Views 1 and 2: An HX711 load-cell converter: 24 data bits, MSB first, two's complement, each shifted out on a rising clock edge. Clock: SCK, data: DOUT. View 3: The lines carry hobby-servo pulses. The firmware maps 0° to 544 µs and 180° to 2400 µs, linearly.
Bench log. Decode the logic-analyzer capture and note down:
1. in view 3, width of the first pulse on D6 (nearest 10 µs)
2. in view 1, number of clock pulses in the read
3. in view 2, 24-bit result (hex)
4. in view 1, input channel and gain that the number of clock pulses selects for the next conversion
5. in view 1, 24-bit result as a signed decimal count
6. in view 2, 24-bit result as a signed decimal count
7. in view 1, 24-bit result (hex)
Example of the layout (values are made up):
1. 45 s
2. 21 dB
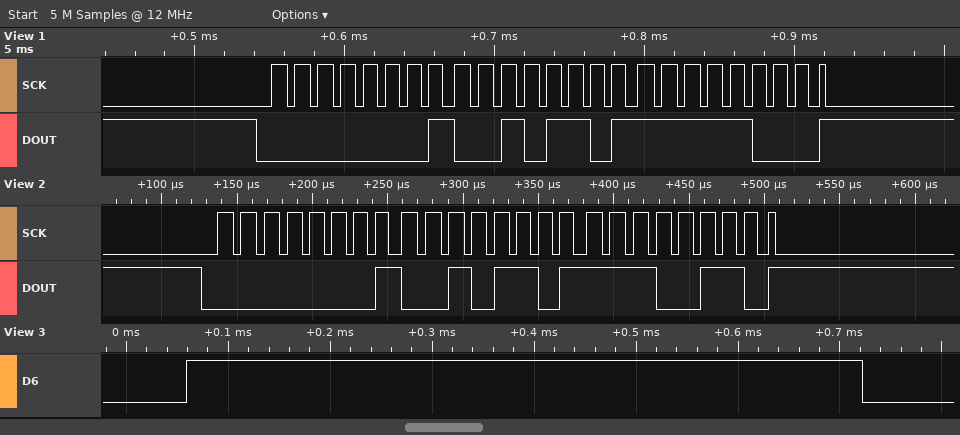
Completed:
1. 660 µs
2. 25
3. 0x012DE6
4. channel A, gain 128
5. 77304
6. 77286
7. 0x012DF8
